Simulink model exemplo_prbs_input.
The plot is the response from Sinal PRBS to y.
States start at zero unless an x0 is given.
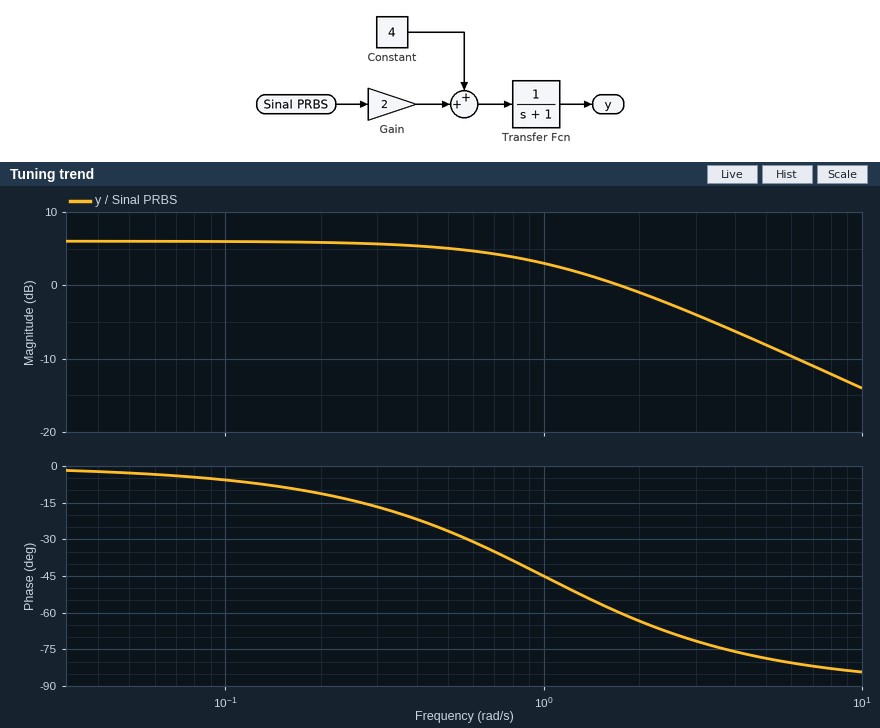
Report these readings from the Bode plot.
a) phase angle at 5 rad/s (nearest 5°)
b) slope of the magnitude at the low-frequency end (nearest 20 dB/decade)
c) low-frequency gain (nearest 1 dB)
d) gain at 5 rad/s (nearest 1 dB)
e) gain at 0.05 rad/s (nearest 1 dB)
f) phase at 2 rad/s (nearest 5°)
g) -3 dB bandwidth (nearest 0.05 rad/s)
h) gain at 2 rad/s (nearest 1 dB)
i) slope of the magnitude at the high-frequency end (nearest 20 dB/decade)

-80°
0 dB/decade
6 dB
-8 dB
6 dB
-65°
1.00 rad/s
-1 dB
-20 dB/decade
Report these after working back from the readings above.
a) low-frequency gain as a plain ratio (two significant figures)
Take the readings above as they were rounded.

2.0
